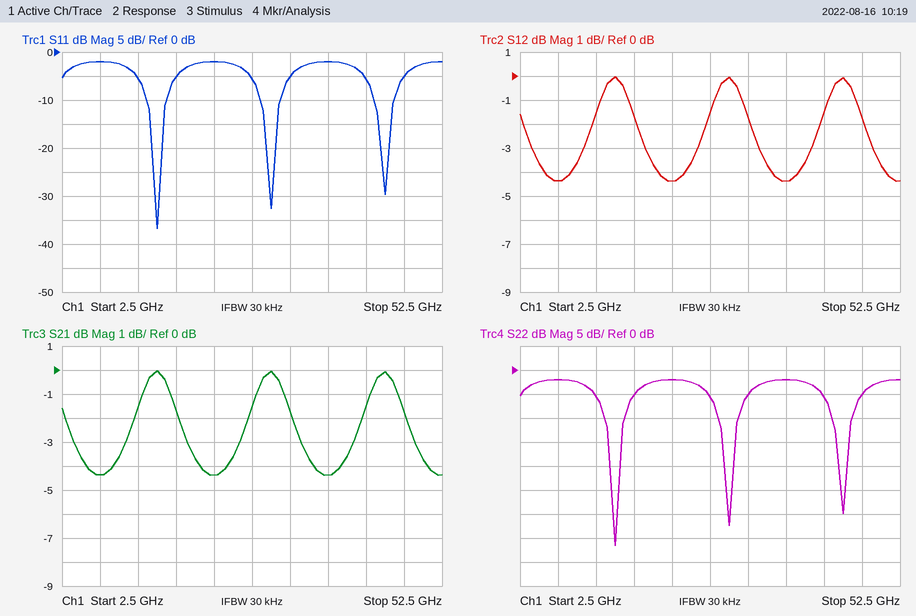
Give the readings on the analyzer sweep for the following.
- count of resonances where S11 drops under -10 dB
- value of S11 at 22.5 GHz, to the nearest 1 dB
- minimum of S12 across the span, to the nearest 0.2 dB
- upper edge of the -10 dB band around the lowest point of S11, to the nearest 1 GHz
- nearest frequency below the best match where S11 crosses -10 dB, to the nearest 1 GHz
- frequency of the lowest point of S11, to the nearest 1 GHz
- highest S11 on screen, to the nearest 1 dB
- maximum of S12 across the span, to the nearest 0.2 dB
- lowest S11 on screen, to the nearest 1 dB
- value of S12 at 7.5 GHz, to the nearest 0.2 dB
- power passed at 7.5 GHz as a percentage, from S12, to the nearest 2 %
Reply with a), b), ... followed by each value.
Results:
a) 3
b) -2 dB
c) -4.4 dB
d) 16 GHz
e) 14 GHz
f) 15 GHz
g) -2 dB
h) 0.0 dB
i) -37 dB
j) -4.4 dB
k) 36 %
